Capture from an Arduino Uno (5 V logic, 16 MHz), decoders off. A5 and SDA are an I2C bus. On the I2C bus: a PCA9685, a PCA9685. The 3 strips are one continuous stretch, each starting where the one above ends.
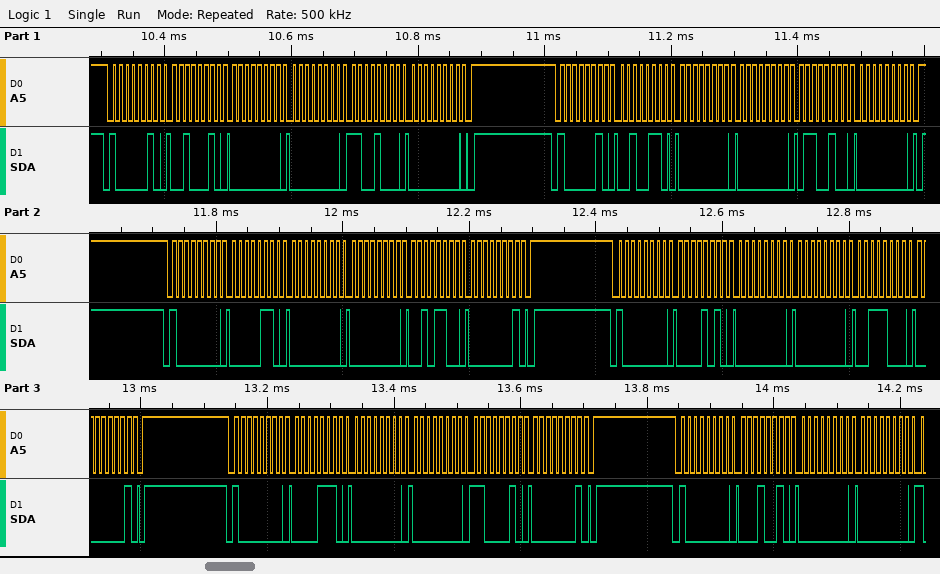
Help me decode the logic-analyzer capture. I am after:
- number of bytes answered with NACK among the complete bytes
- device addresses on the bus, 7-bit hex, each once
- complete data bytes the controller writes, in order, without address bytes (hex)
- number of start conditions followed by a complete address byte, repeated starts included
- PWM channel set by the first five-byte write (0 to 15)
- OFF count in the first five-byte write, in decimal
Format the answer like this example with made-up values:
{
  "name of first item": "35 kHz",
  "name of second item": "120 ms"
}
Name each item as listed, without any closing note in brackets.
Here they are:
{
  "number of bytes answered with NACK among the complete bytes": "0",
  "device addresses on the bus, 7-bit hex, each once": "0x41 0x40",
  "complete data bytes the controller writes, in order, without address bytes": "22 00 00 C8 00 26 00 00 64 00 06 00 00 2C 01 0A 00 00 38 01 0E 00 00 C2 01 12 00 00",
  "number of start conditions followed by a complete address byte, repeated starts included": "6",
  "PWM channel set by the first five-byte write": "7",
  "OFF count in the first five-byte write, in decimal": "200"
}
